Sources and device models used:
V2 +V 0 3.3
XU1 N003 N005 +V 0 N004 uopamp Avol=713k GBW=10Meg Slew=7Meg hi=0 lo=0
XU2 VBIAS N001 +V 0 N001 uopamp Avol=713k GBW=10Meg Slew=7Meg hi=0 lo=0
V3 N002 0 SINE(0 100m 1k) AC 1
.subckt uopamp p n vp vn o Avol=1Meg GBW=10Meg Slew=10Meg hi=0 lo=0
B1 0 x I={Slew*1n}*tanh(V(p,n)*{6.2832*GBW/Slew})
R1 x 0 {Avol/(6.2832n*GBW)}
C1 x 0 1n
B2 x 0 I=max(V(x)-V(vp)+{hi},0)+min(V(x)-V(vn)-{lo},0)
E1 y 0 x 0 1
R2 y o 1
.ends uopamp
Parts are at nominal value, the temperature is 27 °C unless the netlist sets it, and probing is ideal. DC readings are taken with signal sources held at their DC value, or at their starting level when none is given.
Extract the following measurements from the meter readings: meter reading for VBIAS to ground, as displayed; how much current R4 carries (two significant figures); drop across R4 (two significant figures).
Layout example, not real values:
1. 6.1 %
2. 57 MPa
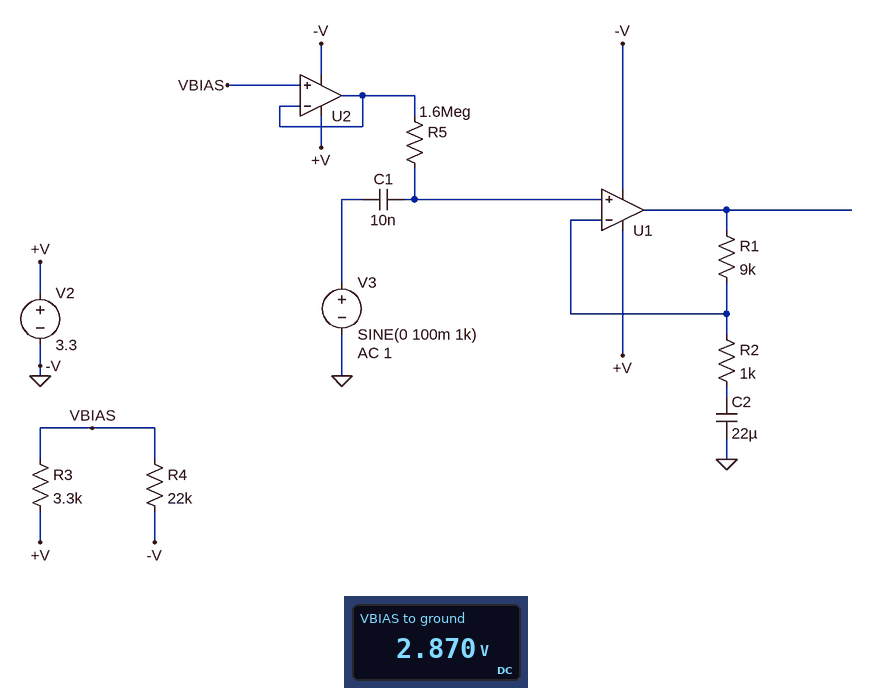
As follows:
1. 2.870 V
2. 130 µA
3. 2.9 V
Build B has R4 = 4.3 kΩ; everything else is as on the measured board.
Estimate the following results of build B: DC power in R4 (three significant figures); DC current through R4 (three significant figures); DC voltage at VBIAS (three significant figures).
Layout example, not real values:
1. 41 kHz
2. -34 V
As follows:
1. 811 µW
2. 434 µA
3. 1.87 V
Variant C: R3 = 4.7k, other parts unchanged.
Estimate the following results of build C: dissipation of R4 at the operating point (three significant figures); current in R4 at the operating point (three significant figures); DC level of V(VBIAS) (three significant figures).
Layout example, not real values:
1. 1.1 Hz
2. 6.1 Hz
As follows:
1. 336 µW
2. 124 µA
3. 2.72 V
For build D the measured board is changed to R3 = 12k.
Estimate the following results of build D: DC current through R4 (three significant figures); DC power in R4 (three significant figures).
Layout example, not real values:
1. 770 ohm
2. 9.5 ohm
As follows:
1. 97.1 µA
2. 207 µW
